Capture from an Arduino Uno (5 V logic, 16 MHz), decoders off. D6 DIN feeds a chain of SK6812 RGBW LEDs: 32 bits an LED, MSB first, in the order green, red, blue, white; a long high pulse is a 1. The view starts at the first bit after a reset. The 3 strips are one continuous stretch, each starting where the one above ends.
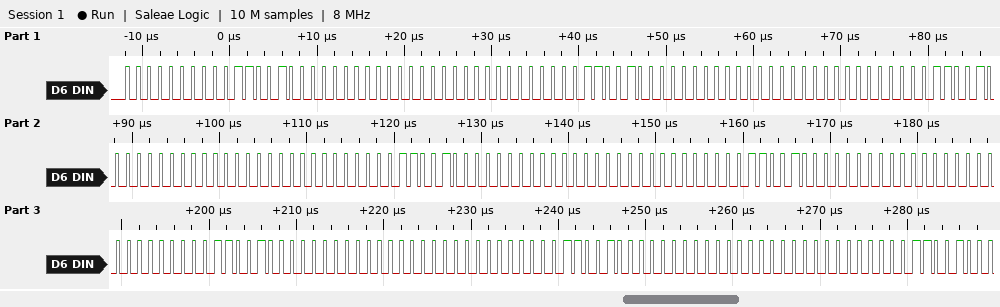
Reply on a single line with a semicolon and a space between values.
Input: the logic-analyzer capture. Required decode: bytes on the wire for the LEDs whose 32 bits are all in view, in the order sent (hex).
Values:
00 32 00 00 00 32 00 00 00 32 00 00 00 32 00 00 00 32 00 00 00 32 00 00 00 32 00 00
